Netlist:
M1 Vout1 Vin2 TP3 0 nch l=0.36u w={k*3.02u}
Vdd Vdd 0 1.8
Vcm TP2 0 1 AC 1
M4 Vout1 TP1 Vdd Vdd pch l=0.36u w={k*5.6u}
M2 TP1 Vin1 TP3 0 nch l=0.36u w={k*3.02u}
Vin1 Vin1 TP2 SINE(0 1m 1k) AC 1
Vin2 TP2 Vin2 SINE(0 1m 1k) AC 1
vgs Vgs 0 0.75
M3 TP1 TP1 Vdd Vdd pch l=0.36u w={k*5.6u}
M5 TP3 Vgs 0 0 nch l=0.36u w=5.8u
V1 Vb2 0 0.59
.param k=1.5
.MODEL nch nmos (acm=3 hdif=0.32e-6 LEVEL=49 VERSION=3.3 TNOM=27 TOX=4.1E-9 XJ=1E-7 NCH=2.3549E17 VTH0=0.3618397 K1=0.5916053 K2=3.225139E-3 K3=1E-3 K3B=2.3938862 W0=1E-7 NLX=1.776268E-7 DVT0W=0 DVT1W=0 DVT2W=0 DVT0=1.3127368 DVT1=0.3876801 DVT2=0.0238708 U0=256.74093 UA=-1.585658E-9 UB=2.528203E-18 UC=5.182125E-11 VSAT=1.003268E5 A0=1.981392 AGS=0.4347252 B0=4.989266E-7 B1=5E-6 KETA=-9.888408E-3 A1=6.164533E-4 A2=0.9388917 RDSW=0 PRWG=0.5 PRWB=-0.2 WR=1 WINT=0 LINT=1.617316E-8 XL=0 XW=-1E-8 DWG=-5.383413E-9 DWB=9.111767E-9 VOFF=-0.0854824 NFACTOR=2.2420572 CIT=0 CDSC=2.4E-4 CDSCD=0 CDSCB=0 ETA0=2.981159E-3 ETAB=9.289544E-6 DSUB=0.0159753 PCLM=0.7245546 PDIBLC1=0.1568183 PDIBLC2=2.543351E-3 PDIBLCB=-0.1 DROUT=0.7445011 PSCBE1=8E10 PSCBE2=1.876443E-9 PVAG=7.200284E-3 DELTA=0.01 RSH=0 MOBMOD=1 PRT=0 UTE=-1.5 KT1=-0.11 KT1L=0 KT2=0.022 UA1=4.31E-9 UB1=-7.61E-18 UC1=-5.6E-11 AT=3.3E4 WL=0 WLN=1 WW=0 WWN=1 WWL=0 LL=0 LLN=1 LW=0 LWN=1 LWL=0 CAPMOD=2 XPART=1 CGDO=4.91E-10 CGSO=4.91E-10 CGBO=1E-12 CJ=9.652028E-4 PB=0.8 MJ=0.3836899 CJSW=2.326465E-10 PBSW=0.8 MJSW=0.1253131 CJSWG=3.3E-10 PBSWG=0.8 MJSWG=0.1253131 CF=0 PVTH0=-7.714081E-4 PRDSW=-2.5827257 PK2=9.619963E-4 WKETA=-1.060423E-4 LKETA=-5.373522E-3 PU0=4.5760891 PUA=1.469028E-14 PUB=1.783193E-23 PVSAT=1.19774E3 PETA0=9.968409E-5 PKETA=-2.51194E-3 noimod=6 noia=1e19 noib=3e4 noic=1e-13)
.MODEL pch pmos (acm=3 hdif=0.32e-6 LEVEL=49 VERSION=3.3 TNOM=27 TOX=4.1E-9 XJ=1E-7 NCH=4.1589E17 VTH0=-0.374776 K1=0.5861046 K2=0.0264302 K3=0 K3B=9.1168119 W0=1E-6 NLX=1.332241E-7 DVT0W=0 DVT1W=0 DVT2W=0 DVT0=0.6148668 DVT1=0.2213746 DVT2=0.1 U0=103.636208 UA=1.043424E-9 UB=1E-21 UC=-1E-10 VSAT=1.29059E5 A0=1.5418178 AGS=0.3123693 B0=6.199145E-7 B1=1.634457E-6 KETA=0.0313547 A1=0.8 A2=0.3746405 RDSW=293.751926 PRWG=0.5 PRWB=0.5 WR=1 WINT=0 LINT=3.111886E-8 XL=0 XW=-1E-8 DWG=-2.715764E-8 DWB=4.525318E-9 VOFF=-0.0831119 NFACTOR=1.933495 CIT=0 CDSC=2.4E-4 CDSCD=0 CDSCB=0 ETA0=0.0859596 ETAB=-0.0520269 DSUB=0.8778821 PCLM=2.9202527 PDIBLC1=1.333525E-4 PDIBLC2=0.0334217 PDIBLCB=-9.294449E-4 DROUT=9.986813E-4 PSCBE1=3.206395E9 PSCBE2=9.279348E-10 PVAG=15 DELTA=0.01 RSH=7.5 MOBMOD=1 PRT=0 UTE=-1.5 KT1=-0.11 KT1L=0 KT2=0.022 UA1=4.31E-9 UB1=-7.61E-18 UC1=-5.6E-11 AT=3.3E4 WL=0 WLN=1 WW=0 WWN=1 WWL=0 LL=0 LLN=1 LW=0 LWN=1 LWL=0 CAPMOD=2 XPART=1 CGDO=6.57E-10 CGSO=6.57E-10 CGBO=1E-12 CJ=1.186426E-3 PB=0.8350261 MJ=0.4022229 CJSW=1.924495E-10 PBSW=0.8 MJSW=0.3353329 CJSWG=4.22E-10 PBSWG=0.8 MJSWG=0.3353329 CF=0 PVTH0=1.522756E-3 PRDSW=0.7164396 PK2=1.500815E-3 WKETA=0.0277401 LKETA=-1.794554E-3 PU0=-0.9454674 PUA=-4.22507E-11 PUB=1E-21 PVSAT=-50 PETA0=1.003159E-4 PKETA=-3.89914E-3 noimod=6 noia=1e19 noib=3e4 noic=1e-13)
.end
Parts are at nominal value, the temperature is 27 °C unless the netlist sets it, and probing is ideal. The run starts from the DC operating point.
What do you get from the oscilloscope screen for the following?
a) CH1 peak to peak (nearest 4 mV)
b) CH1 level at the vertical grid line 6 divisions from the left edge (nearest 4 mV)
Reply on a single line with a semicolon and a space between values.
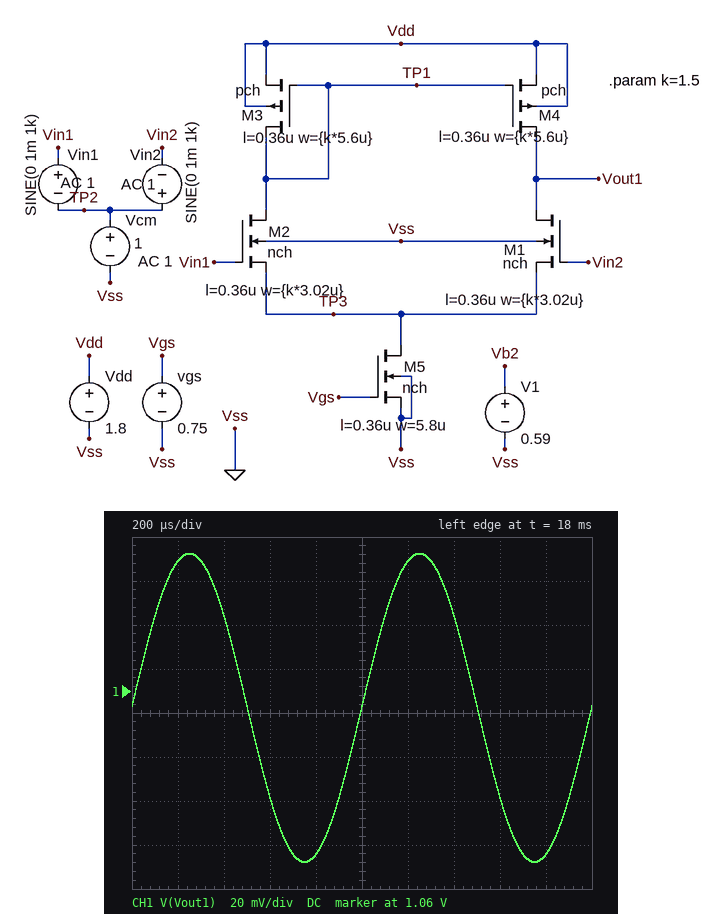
140 mV; 1.120 V
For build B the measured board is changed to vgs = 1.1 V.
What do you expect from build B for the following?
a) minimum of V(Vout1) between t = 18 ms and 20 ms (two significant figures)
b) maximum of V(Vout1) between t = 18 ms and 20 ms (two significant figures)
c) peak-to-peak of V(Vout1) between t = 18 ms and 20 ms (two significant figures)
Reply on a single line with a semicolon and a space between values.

810 mV; 920 mV; 110 mV
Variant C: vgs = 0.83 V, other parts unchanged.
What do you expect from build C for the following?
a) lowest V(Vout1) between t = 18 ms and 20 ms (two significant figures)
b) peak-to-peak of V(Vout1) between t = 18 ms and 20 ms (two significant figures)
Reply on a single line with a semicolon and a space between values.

920 mV; 130 mV
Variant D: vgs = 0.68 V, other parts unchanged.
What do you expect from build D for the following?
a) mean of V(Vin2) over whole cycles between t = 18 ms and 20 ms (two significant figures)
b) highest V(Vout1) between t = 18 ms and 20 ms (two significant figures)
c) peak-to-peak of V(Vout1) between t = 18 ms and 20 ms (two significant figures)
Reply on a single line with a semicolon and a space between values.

1.0 V; 1.2 V; 150 mV
